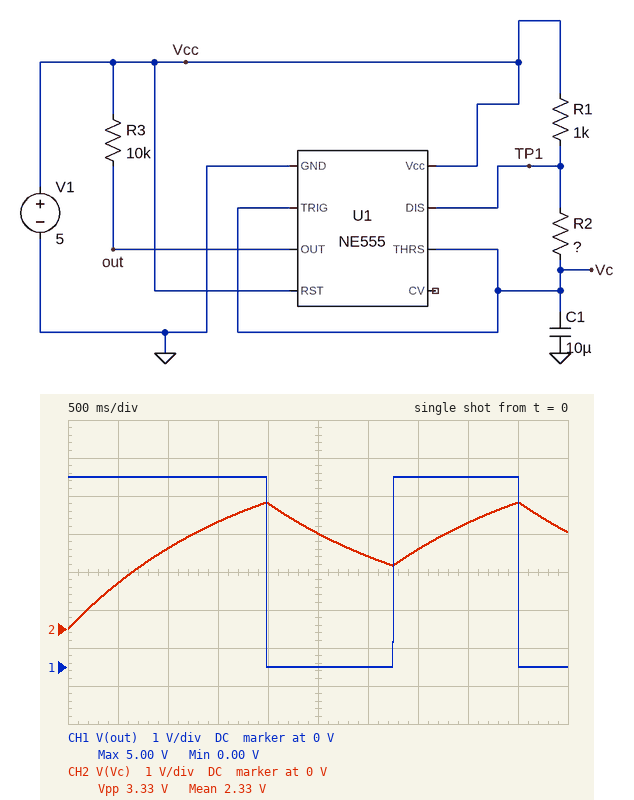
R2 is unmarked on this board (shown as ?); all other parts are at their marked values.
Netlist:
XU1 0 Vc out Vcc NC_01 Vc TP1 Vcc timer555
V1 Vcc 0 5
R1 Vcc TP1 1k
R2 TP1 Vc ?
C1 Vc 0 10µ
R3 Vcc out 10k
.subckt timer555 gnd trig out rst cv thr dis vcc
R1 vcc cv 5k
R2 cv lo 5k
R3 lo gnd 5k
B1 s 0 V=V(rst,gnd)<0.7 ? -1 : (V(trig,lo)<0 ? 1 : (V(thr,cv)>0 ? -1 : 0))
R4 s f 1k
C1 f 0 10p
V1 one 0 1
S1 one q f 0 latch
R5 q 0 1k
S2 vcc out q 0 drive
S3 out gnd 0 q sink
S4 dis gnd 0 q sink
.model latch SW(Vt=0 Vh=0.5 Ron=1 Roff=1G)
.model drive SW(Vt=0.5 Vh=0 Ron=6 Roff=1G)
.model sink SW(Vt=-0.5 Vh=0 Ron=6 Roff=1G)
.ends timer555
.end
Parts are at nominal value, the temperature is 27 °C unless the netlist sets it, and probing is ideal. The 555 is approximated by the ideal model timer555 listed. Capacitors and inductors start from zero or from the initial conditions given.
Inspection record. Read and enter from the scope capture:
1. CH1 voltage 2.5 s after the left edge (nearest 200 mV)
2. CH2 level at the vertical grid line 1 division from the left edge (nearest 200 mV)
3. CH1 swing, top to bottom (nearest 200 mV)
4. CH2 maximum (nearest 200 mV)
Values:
0 V
1.2 V
5.0 V
3.4 V
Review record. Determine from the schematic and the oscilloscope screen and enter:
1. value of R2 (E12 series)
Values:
180 kΩ
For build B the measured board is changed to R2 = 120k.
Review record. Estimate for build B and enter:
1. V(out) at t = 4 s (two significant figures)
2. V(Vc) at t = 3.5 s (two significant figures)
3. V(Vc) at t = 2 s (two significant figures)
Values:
5.0 V
2.2 V
1.9 V
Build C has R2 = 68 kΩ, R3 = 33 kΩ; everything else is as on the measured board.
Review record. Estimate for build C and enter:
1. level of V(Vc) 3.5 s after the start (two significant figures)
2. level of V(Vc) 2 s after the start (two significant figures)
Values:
3.0 V
2.2 V
